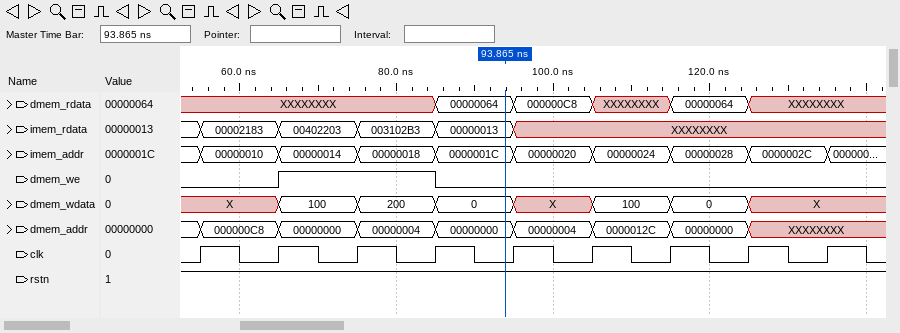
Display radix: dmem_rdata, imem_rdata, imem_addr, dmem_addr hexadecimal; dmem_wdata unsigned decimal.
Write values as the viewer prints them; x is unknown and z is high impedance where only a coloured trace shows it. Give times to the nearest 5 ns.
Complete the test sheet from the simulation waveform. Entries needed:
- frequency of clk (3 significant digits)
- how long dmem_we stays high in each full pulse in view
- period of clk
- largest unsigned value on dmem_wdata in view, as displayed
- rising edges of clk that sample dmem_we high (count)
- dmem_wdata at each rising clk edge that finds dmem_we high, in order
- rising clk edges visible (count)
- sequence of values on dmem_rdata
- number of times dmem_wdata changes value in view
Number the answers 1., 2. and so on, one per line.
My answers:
1. 100 MHz
2. 20 ns
3. 10 ns
4. 200
5. 2
6. 100, 200
7. 9
8. XXXXXXXX, 00000064, 000000C8, XXXXXXXX, 00000064, XXXXXXXX
9. 7
